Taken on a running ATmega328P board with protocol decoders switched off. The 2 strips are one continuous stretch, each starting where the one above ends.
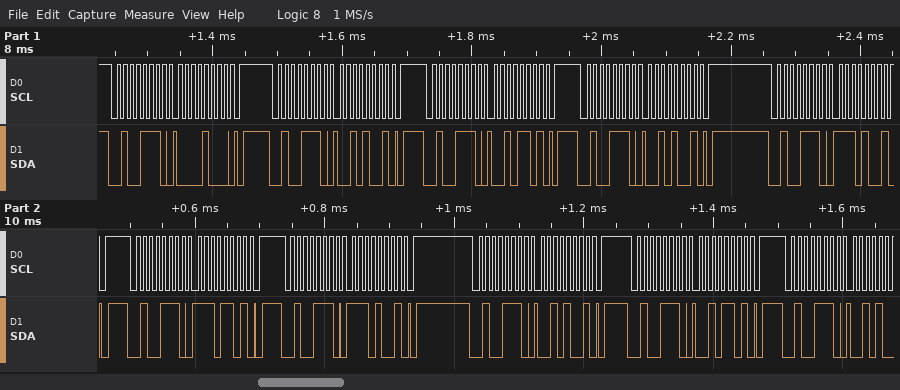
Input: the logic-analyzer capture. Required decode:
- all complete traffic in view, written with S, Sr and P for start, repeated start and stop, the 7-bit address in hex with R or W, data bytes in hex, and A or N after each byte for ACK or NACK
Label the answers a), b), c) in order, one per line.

a) S 27W A 08 A P S 27W A 29 A P S 27W A 2D A P S 27W A 29 A P S 27W A E9 A P S 27W A ED A P S 27W A E9 A P S 27W A 29 A P S 27W A 2D A P S 27W A
